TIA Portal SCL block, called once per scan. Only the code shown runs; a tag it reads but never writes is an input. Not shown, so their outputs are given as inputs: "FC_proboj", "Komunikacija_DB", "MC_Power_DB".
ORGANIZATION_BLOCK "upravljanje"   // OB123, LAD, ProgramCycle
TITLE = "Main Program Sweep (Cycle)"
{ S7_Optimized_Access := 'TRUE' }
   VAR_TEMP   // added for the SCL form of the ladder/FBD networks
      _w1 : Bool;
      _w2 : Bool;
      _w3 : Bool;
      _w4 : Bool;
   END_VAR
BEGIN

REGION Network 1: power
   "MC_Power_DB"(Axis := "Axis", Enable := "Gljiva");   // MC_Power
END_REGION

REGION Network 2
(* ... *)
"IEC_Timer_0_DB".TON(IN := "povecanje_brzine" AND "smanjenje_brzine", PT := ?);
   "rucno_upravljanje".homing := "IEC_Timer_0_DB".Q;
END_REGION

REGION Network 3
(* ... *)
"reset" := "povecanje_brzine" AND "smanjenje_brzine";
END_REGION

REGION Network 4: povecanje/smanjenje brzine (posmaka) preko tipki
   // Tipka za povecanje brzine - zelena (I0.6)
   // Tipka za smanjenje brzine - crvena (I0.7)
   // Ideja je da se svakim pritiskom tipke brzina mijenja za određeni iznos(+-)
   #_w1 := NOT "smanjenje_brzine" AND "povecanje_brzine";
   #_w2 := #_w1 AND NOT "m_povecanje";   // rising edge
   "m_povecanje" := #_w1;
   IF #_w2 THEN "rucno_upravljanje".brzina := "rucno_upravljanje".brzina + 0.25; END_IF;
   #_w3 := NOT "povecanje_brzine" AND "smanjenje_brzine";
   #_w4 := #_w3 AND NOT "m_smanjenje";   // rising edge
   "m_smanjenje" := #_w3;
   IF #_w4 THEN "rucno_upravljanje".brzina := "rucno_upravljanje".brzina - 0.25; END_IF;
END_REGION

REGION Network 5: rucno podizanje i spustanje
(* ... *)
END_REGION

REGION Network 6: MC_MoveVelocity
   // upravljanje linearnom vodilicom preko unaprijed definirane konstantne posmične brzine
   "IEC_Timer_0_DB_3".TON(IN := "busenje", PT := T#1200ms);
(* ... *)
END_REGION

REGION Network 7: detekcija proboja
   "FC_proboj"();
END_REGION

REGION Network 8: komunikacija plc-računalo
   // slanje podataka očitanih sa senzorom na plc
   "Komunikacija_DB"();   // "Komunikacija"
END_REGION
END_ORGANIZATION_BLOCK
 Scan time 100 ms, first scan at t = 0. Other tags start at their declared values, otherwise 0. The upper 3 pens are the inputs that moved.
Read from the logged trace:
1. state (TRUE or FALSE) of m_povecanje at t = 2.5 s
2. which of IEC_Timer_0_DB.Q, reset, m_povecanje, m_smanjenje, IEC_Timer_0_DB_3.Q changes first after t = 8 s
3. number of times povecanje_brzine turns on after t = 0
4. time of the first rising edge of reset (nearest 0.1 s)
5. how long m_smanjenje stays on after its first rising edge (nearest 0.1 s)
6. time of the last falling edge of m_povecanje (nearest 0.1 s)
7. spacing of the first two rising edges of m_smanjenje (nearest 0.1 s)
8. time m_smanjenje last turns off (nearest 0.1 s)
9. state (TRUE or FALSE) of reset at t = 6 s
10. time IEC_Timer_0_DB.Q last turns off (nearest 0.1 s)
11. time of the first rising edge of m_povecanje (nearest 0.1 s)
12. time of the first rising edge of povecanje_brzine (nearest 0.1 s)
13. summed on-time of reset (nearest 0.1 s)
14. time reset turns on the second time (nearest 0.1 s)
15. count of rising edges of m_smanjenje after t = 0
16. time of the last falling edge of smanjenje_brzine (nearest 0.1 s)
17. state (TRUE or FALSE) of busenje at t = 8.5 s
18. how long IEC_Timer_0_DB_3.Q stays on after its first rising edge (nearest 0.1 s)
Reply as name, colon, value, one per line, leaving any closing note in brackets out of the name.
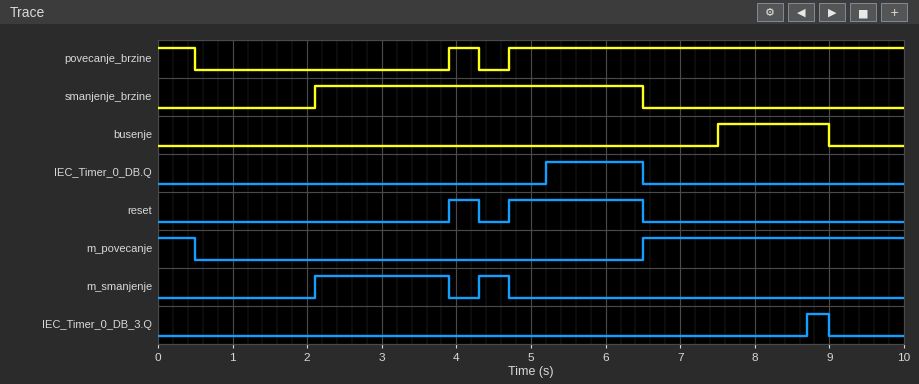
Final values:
state (TRUE or FALSE) of m_povecanje at t = 2.5 s: FALSE
which of IEC_Timer_0_DB.Q, reset, m_povecanje, m_smanjenje, IEC_Timer_0_DB_3.Q changes first after t = 8 s: IEC_Timer_0_DB_3.Q
number of times povecanje_brzine turns on after t = 0: 2
time of the first rising edge of reset: 3.9 s
how long m_smanjenje stays on after its first rising edge: 1.8 s
time of the last falling edge of m_povecanje: 0.5 s
spacing of the first two rising edges of m_smanjenje: 2.2 s
time m_smanjenje last turns off: 4.7 s
state (TRUE or FALSE) of reset at t = 6 s: TRUE
time IEC_Timer_0_DB.Q last turns off: 6.5 s
time of the first rising edge of m_povecanje: 6.5 s
time of the first rising edge of povecanje_brzine: 3.9 s
summed on-time of reset: 2.2 s
time reset turns on the second time: 4.7 s
count of rising edges of m_smanjenje after t = 0: 2
time of the last falling edge of smanjenje_brzine: 6.5 s
state (TRUE or FALSE) of busenje at t = 8.5 s: TRUE
how long IEC_Timer_0_DB_3.Q stays on after its first rising edge: 0.3 s
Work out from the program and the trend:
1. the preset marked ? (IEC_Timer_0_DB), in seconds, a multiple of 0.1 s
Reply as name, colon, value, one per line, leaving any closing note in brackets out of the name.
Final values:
the preset marked ? (IEC_Timer_0_DB), in seconds, a multiple of 0.1 s: 0.5 s
